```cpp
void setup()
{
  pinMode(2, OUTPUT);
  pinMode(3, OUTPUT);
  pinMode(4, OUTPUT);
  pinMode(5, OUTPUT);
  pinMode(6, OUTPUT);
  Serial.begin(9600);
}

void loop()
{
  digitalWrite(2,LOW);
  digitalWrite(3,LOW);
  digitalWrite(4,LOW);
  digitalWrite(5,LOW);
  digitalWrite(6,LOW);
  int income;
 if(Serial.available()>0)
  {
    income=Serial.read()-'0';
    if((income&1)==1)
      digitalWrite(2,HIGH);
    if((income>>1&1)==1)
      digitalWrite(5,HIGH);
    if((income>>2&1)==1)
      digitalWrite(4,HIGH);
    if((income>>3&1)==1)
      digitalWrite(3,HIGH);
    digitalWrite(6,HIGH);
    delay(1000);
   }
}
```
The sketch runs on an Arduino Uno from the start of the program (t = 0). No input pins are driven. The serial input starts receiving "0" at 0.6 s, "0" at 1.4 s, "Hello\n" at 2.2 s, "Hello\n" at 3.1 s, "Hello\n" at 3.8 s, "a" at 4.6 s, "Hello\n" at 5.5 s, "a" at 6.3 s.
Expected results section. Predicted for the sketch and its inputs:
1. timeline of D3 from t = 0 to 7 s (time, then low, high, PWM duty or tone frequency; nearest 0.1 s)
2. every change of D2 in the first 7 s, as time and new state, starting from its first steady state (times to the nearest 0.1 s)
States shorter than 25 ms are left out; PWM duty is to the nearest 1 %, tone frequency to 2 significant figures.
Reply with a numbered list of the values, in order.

1. 0 s low; 2.6 s high; 3.6 s low; 4.6 s high
2. 0 s low; 3.6 s high; 4.6 s low; 6.6 s high
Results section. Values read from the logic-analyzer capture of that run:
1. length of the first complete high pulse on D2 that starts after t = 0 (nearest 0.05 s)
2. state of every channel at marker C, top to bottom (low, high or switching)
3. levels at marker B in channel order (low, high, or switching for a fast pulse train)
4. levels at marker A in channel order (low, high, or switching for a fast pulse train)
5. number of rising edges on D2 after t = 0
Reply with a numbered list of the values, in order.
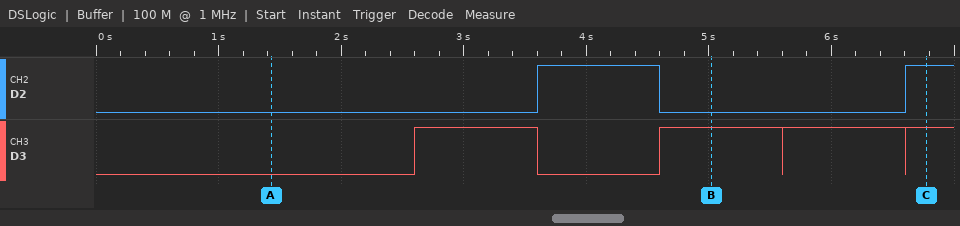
1. 1.00 s
2. D2 high, D3 high
3. D2 low, D3 high
4. D2 low, D3 low
5. 2
